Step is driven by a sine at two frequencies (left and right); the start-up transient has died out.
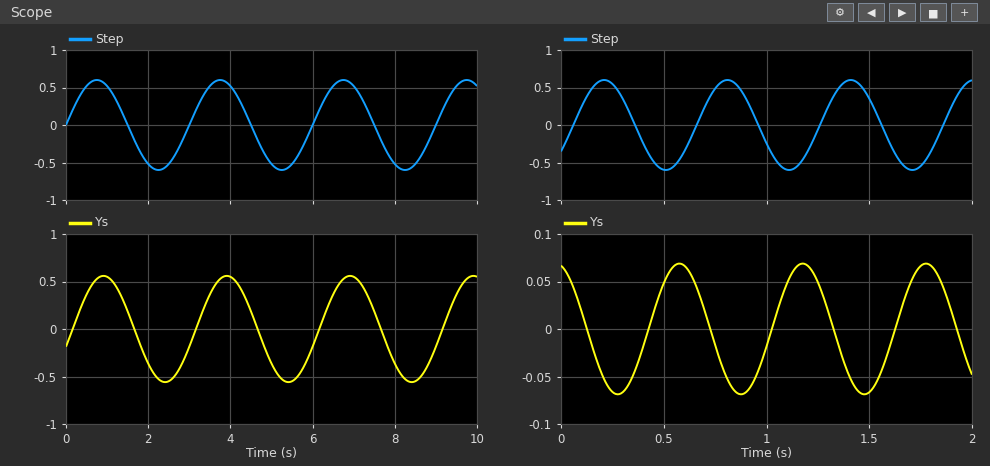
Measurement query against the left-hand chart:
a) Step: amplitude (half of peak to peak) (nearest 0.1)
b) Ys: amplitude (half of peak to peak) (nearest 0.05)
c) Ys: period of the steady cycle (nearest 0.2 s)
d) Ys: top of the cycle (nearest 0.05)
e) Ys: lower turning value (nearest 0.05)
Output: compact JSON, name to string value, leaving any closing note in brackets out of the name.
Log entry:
{"Step: amplitude (half of peak to peak)": "0.6", "Ys: amplitude (half of peak to peak)": "0.55", "Ys: period of the steady cycle": "3.0 s", "Ys: top of the cycle": "0.55", "Ys: lower turning value": "-0.55"}
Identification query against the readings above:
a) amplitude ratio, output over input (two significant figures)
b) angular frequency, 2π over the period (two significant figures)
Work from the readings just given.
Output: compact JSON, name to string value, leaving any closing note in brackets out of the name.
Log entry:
{"amplitude ratio, output over input": "0.92", "angular frequency, 2π over the period": "2.1 rad/s"}
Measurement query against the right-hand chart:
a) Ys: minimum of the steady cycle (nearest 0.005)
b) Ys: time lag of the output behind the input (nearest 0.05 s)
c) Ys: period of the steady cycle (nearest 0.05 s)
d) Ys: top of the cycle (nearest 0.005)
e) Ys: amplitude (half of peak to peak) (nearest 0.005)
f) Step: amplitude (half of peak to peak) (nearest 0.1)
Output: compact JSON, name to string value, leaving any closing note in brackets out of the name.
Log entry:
{"Ys: minimum of the steady cycle": "-0.070", "Ys: time lag of the output behind the input": "0.35 s", "Ys: period of the steady cycle": "0.60 s", "Ys: top of the cycle": "0.070", "Ys: amplitude (half of peak to peak)": "0.070", "Step: amplitude (half of peak to peak)": "0.6"}
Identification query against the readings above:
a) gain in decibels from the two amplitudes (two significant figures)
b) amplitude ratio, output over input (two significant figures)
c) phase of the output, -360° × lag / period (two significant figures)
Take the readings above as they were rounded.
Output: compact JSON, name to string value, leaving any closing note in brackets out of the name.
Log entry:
{"gain in decibels from the two amplitudes": "-19 dB", "amplitude ratio, output over input": "0.12", "phase of the output, -360° × lag / period": "-210°"}
